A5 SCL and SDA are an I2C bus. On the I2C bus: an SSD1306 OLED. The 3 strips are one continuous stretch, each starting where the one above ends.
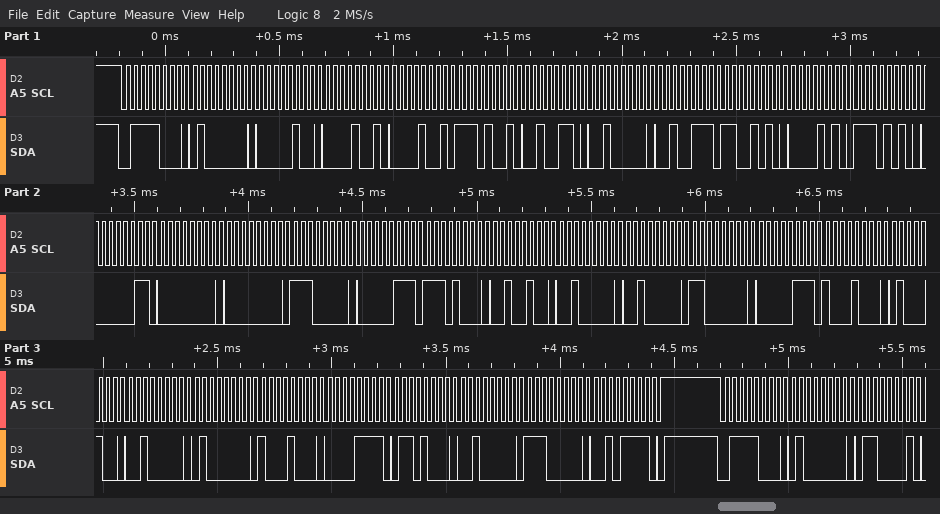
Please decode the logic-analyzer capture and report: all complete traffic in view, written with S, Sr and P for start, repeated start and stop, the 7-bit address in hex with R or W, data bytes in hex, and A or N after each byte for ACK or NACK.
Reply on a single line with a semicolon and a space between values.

S 3CW A 40 A 04 A 09 A 09 A E9 A 26 A 20 A 27 A CA A 0A A EA A 03 A 00 A 00 A E0 A 07 A E8 A 24 A 20 A 20 A C0 A 07 A 88 A 44 A 20 A 40 A 88 A 0F A 68 A 20 A E0 A 2F A P S 3CW A 40 A 61 A
